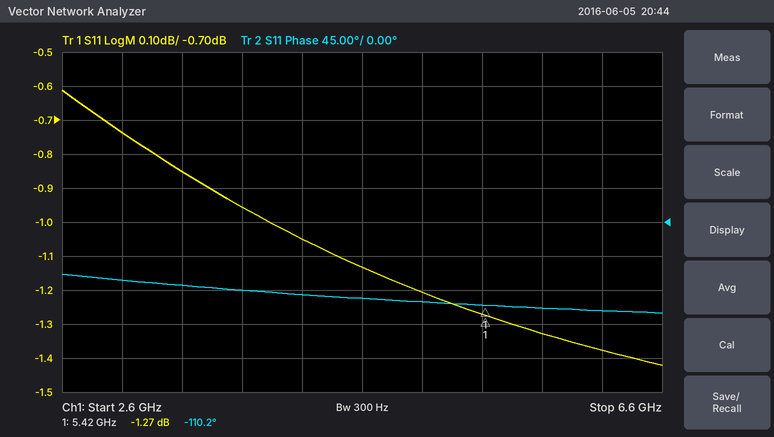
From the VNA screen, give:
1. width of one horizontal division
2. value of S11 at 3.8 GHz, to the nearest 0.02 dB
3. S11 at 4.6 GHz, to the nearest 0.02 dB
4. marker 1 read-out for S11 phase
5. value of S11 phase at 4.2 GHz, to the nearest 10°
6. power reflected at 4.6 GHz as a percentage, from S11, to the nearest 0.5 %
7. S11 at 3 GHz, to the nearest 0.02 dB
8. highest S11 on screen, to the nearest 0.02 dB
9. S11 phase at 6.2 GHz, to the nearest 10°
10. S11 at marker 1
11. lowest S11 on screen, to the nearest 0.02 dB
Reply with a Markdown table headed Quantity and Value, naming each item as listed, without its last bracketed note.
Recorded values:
| Quantity | Value |
|---|---|
| width of one horizontal division | 400 MHz |
| value of S11 at 3.8 GHz, to the nearest 0.02 dB | -0.96 dB |
| S11 at 4.6 GHz, to the nearest 0.02 dB | -1.14 dB |
| marker 1 read-out for S11 phase | -110.2° |
| value of S11 phase at 4.2 GHz, to the nearest 10° | -100° |
| power reflected at 4.6 GHz as a percentage, from S11, to the nearest 0.5 % | 77.0 % |
| S11 at 3 GHz, to the nearest 0.02 dB | -0.74 dB |
| highest S11 on screen, to the nearest 0.02 dB | -0.62 dB |
| S11 phase at 6.2 GHz, to the nearest 10° | -120° |
| S11 at marker 1 | -1.27 dB |
| lowest S11 on screen, to the nearest 0.02 dB | -1.42 dB |
